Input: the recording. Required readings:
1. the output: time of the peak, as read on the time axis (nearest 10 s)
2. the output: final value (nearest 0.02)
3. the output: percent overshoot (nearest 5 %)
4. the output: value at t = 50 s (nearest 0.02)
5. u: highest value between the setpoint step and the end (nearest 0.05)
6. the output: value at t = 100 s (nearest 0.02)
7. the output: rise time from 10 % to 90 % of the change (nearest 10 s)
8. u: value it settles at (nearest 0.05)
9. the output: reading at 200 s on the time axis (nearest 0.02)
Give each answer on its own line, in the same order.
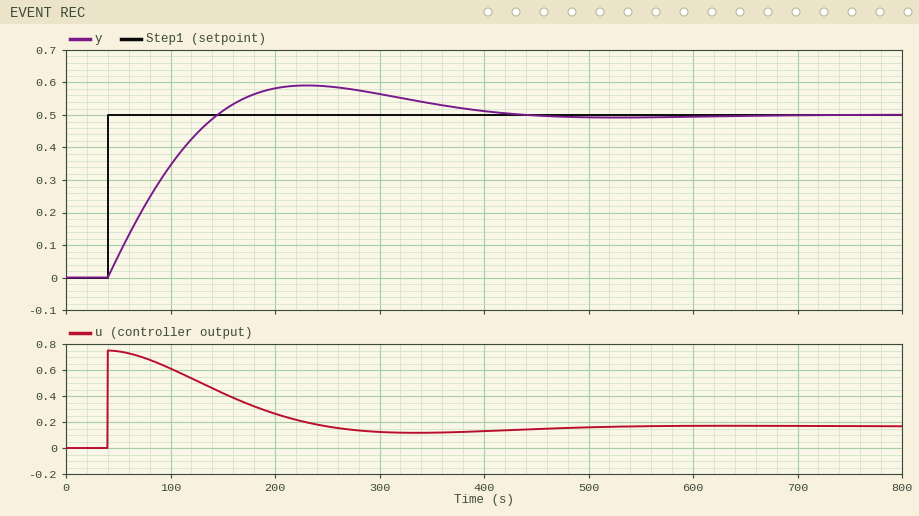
230 s
0.50
20 %
0.06
0.75
0.34
80 s
0.15
0.58
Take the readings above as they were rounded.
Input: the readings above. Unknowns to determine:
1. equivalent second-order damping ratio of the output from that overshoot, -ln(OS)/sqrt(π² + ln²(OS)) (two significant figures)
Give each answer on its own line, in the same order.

0.46
